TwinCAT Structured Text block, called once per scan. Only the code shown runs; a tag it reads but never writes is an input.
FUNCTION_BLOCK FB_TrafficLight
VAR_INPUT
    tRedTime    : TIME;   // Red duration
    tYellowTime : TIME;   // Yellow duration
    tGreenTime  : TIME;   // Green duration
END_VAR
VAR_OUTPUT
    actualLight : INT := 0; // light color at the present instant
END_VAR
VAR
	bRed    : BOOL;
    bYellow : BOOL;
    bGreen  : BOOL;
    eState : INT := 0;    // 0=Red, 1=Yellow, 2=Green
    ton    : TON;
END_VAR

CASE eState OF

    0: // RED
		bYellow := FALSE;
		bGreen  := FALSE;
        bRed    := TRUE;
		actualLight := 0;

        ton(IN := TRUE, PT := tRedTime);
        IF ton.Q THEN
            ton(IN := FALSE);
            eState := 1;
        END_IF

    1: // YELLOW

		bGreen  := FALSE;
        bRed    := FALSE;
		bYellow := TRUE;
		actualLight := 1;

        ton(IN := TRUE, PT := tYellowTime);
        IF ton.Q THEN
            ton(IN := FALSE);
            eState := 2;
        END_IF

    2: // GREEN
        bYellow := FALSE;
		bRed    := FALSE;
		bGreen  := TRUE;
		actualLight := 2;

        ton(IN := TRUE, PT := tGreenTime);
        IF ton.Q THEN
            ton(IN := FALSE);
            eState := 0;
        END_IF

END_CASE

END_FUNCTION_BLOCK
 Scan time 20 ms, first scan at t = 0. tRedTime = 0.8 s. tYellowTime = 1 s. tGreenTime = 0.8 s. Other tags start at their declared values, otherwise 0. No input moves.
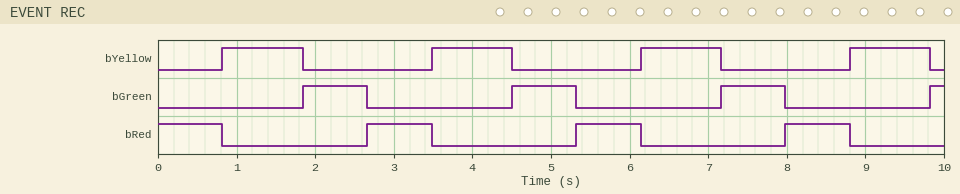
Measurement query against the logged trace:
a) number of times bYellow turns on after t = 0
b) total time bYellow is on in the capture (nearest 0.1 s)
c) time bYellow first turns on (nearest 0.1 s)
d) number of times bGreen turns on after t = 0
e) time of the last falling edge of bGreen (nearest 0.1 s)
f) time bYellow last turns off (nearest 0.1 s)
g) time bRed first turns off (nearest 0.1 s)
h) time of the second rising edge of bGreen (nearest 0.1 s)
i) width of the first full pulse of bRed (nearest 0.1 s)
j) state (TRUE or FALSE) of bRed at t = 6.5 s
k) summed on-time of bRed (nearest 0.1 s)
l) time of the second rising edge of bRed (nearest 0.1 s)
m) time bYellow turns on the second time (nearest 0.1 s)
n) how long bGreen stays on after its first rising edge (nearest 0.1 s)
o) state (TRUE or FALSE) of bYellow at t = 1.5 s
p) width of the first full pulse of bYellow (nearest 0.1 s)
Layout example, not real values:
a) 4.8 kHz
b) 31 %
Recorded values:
a) 4
b) 4.1 s
c) 0.8 s
d) 4
e) 8.0 s
f) 9.8 s
g) 0.8 s
h) 4.5 s
i) 0.8 s
j) FALSE
k) 3.3 s
l) 5.3 s
m) 3.5 s
n) 0.8 s
o) TRUE
p) 1.0 s
